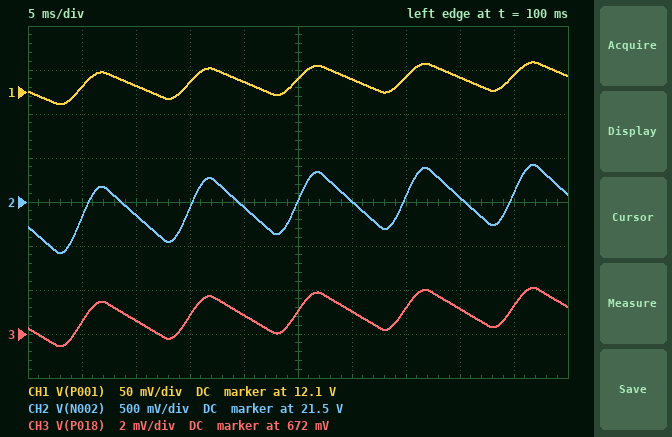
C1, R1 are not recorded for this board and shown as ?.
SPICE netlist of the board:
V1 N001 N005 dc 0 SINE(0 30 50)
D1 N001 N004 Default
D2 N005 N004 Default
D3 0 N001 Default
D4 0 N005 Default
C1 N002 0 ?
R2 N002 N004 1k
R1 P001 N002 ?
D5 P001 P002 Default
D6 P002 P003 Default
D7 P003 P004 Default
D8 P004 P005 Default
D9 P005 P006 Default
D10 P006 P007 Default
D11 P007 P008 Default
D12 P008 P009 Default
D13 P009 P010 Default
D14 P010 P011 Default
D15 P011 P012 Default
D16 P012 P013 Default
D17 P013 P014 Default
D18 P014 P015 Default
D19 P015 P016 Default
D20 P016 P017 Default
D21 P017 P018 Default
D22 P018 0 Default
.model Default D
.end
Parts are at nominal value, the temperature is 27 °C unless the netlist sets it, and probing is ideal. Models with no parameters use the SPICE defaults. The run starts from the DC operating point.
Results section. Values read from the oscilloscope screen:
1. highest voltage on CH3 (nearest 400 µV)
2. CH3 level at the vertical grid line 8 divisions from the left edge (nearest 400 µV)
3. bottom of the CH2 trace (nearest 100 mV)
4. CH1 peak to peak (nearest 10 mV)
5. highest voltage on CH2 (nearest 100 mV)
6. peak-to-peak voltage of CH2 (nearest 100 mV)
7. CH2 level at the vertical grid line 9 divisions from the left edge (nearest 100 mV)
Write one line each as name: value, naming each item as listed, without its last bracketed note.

highest voltage on CH3: 674.0 mV
CH3 level at the vertical grid line 8 divisions from the left edge: 673.2 mV
bottom of the CH2 trace: 20.9 V
CH1 peak to peak: 50 mV
highest voltage on CH2: 21.9 V
peak-to-peak voltage of CH2: 1.0 V
CH2 level at the vertical grid line 9 divisions from the left edge: 21.6 V
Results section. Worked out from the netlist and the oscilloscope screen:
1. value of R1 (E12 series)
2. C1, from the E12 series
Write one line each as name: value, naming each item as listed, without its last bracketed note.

value of R1: 4.7 kΩ
C1, from the E12 series: 18 µF
